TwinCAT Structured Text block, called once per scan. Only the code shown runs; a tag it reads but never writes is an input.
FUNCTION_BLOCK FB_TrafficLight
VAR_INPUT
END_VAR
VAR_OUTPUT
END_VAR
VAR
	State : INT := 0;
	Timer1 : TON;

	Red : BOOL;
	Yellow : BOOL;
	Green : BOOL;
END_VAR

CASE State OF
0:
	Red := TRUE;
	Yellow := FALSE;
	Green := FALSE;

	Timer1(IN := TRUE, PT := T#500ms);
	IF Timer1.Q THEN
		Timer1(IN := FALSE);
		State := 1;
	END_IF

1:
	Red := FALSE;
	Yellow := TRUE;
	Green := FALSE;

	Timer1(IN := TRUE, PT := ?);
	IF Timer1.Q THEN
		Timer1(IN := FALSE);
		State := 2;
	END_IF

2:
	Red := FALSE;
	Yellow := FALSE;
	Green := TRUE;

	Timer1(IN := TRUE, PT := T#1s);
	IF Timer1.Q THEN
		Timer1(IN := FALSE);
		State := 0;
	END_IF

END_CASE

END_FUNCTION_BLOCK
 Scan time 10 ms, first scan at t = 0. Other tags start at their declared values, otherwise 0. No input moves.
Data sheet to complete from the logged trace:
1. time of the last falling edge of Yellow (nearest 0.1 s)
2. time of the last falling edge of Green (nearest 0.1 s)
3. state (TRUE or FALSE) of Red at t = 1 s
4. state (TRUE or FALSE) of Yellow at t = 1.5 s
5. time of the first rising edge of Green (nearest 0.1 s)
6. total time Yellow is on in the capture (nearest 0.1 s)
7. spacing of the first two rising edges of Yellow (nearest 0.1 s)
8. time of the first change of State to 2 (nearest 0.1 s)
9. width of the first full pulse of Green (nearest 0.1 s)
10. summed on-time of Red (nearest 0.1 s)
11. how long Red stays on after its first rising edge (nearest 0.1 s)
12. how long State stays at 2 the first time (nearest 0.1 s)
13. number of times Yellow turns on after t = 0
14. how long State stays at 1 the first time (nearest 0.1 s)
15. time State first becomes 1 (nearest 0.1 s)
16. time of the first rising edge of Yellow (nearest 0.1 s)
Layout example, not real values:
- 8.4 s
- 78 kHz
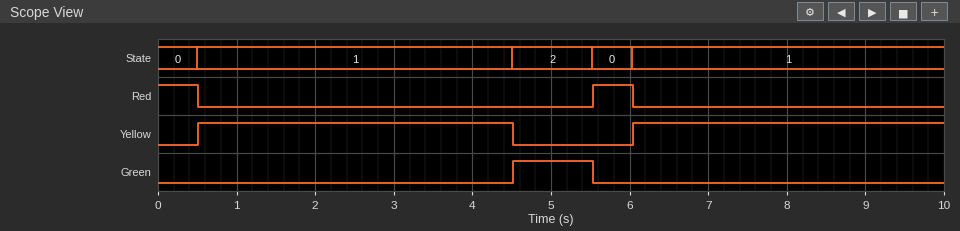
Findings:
- 4.5 s
- 5.5 s
- FALSE
- TRUE
- 4.5 s
- 8.0 s
- 5.5 s
- 4.5 s
- 1.0 s
- 1.0 s
- 0.5 s
- 1.0 s
- 2
- 4.0 s
- 0.5 s
- 0.5 s
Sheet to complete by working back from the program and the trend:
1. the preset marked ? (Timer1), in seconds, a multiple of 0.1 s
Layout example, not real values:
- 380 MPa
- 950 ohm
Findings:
- 4.0 s
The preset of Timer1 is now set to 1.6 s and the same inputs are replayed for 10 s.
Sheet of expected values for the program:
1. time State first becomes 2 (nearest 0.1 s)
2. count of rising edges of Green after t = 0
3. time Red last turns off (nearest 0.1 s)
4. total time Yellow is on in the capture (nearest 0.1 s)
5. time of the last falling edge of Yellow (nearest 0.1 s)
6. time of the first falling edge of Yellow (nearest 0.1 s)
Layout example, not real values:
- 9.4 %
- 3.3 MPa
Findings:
- 2.1 s
- 3
- 9.9 s
- 4.9 s
- 8.4 s
- 2.1 s
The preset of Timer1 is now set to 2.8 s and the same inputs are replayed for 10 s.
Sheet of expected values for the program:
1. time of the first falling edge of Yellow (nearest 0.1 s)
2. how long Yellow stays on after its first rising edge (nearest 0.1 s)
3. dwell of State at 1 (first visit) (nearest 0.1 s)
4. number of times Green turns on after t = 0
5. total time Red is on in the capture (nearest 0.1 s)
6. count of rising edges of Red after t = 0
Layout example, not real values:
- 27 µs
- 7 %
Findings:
- 3.3 s
- 2.8 s
- 2.8 s
- 2
- 1.5 s
- 2
